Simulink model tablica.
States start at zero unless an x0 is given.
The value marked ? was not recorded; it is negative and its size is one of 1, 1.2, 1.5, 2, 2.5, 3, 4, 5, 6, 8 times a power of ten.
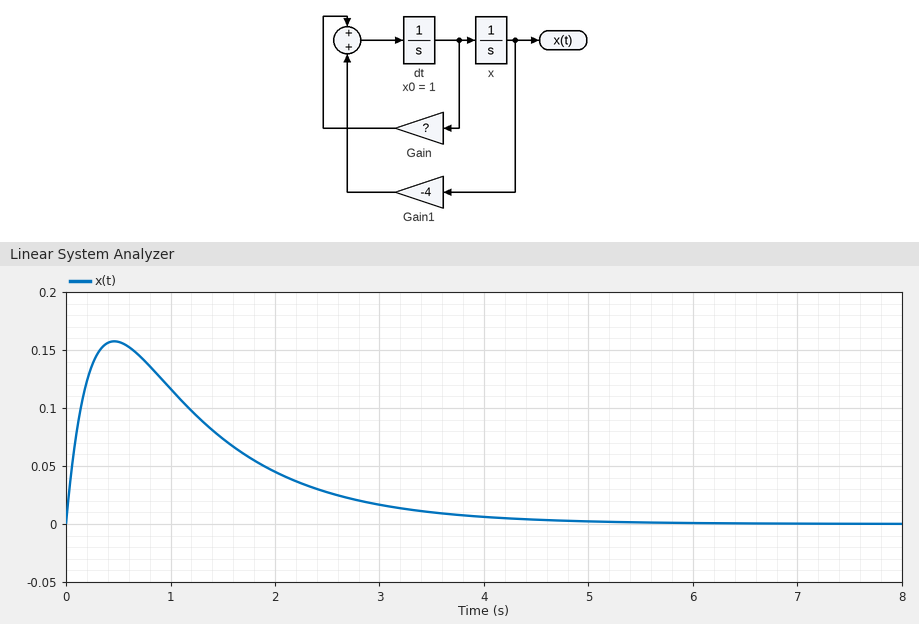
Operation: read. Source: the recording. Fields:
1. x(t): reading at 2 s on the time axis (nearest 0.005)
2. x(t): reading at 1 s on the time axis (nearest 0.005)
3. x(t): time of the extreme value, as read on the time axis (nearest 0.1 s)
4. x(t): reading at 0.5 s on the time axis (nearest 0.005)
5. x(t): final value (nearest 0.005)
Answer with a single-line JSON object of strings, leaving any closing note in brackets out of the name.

{"x(t): reading at 2 s on the time axis": "0.045", "x(t): reading at 1 s on the time axis": "0.115", "x(t): time of the extreme value, as read on the time axis": "0.5 s", "x(t): reading at 0.5 s on the time axis": "0.155", "x(t): final value": "0.000"}
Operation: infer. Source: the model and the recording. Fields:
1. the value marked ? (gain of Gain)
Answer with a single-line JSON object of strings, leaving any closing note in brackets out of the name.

{"the value marked ?": "-5"}
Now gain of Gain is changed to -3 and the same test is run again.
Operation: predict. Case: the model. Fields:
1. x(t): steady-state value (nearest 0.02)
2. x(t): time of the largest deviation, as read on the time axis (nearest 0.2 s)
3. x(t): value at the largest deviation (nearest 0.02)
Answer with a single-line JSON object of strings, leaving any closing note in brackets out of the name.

{"x(t): steady-state value": "0.00", "x(t): time of the largest deviation, as read on the time axis": "0.6 s", "x(t): value at the largest deviation": "0.22"}
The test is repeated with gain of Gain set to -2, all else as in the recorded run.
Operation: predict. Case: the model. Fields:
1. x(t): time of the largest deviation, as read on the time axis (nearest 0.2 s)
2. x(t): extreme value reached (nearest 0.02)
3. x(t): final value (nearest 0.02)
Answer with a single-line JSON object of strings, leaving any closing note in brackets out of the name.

{"x(t): time of the largest deviation, as read on the time axis": "0.6 s", "x(t): extreme value reached": "0.28", "x(t): final value": "0.00"}
